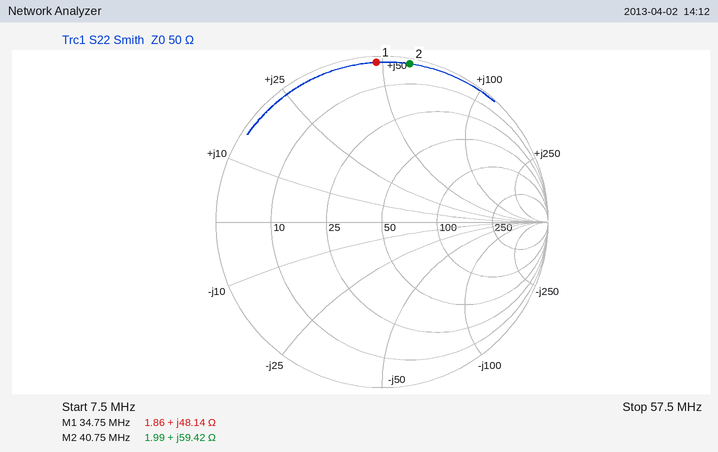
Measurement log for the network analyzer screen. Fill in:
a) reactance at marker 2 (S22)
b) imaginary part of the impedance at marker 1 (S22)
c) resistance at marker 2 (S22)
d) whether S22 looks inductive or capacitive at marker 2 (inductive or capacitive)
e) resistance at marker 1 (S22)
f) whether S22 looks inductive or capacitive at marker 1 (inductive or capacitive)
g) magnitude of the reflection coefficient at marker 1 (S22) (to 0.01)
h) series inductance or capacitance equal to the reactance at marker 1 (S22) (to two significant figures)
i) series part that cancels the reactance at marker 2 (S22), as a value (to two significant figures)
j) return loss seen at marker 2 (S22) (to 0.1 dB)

+59.42 Ω
+48.14 Ω
1.99 Ω
inductive
1.86 Ω
inductive
0.96
220 nH
66 pF
0.3 dB
